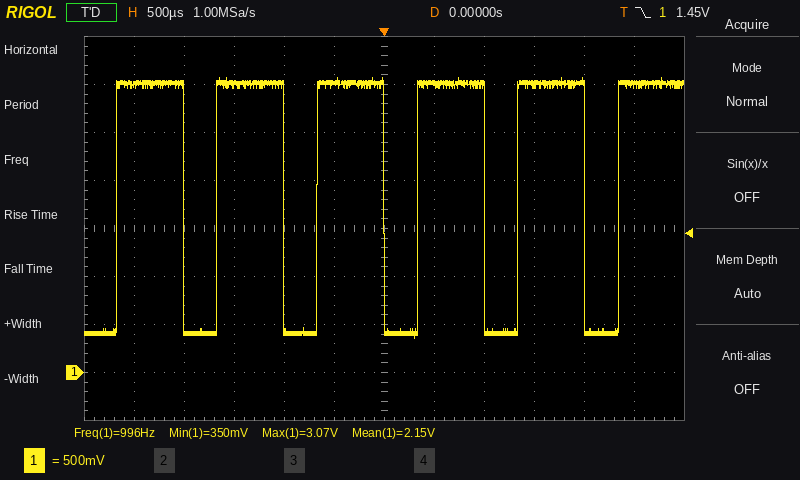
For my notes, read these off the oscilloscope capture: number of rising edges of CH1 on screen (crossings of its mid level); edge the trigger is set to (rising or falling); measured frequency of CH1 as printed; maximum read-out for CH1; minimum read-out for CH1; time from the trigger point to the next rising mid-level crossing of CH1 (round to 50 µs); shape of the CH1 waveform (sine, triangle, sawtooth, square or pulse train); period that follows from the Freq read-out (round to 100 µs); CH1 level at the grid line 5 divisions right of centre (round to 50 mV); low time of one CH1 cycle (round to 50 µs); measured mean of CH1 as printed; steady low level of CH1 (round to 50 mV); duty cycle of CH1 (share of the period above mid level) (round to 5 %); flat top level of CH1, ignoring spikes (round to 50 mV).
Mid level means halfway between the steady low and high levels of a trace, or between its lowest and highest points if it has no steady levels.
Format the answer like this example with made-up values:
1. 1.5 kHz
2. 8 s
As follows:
1. 6
2. falling
3. 996 Hz
4. 3.07 V
5. 350 mV
6. 350 µs
7. pulse train
8. 1.0 ms
9. 3.00 V
10. 350 µs
11. 2.15 V
12. 400 mV
13. 65 %
14. 3.00 V
